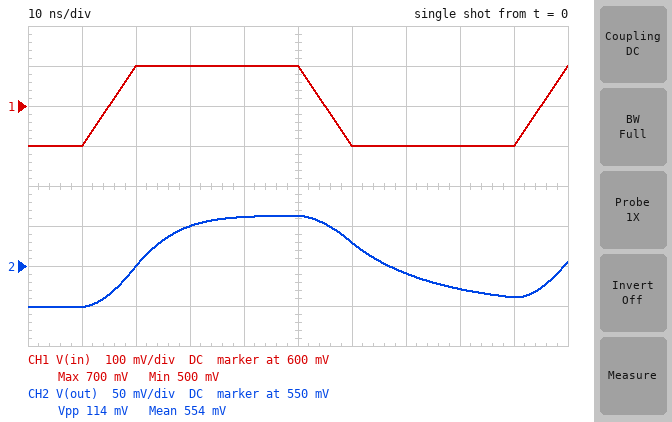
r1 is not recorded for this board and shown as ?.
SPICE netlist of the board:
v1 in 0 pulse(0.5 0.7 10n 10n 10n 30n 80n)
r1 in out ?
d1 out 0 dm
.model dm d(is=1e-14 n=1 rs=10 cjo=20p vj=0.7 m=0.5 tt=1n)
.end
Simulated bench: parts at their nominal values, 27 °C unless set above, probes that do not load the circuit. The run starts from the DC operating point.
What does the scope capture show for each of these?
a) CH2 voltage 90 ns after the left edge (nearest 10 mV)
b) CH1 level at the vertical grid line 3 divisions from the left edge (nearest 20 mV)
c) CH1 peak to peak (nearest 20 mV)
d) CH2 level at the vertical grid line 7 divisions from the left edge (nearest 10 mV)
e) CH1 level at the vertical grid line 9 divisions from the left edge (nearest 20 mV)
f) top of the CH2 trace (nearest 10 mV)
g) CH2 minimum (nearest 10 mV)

510 mV
700 mV
200 mV
540 mV
500 mV
610 mV
500 mV
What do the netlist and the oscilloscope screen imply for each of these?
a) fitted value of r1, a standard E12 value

470 Ω
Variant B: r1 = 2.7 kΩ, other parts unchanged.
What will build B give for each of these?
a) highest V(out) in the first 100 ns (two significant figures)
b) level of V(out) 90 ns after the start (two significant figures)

550 mV
530 mV
